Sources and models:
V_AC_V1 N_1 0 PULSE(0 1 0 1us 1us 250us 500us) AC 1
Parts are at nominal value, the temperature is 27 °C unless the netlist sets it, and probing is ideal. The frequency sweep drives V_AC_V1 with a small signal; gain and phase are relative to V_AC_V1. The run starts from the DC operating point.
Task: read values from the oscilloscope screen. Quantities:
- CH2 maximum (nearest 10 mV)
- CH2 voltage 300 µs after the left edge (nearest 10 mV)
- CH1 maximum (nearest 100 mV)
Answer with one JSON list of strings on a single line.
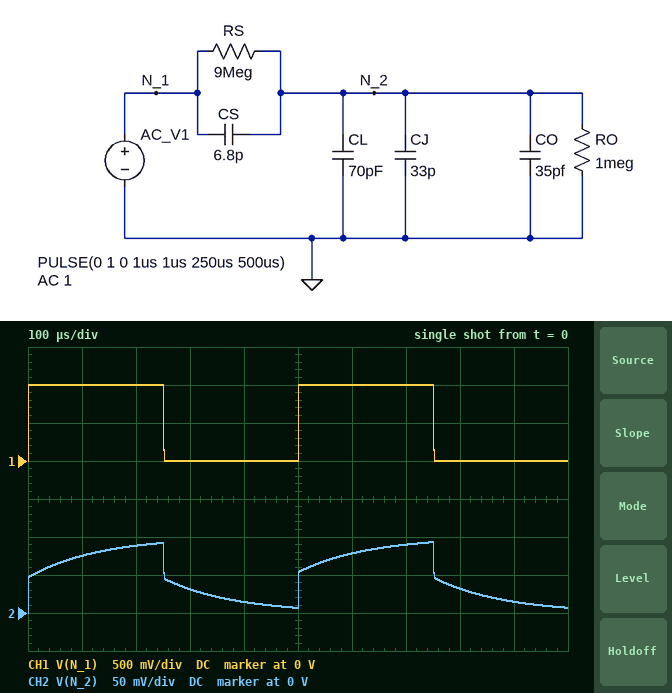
["90 mV", "30 mV", "1.0 V"]
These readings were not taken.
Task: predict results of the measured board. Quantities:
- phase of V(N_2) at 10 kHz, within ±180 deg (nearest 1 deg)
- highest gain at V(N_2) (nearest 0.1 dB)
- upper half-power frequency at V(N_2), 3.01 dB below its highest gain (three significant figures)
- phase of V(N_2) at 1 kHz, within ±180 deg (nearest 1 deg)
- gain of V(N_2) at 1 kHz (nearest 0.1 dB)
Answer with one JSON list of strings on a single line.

["-8 deg", "-20.0 dB", "1.63 kHz", "-18 deg", "-21.6 dB"]
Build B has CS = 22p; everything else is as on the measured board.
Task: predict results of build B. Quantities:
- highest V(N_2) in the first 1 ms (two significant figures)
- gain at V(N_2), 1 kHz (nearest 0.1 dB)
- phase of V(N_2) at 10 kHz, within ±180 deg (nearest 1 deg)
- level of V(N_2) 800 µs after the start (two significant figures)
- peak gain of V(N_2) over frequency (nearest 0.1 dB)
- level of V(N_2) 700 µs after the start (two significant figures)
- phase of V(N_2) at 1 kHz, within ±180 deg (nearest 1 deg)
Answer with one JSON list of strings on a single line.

["140 mV", "-18.5 dB", "2 deg", "-23 mV", "-17.2 dB", "110 mV", "9 deg"]
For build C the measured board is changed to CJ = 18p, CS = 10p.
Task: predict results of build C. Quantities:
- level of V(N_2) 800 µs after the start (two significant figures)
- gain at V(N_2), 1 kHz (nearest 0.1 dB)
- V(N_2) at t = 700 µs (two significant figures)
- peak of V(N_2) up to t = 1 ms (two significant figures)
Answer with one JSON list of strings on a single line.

["15 mV", "-20.7 dB", "96 mV", "97 mV"]
